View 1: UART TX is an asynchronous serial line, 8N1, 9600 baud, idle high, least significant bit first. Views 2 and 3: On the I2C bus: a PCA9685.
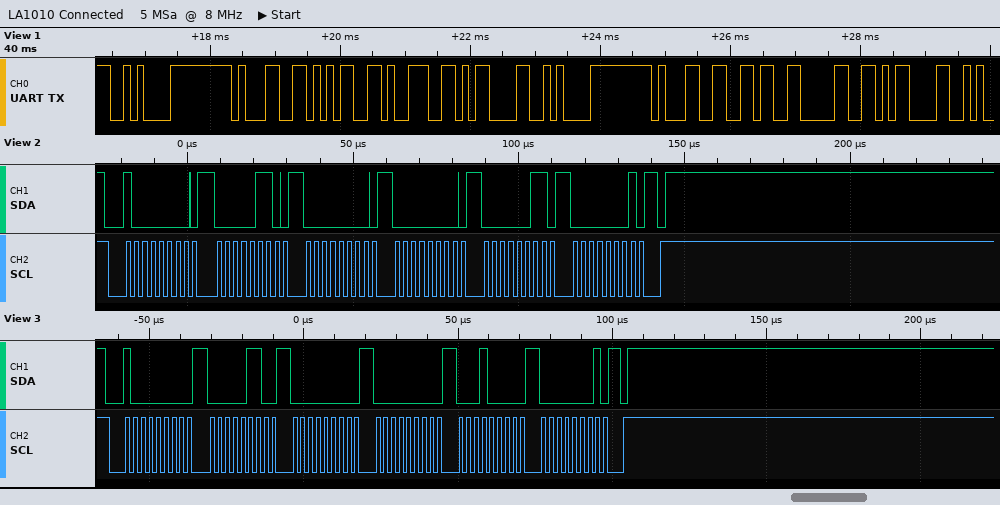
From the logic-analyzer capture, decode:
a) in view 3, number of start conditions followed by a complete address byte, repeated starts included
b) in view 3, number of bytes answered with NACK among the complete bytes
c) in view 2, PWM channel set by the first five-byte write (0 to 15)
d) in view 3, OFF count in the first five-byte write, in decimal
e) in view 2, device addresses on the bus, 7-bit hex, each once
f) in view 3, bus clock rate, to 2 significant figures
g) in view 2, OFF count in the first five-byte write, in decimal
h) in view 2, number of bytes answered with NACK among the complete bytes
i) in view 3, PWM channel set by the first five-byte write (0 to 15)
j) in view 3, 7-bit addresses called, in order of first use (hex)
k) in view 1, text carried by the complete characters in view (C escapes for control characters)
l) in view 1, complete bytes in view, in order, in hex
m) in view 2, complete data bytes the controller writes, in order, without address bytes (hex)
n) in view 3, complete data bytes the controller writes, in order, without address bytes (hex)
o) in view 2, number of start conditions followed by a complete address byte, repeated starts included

1
0
0
272
0x40
400 kHz
259
0
0
0x40
"\n159\r\n160\r"
0A 31 35 39 0D 0A 31 36 30 0D
06 00 00 03 01
06 00 00 10 01
1
